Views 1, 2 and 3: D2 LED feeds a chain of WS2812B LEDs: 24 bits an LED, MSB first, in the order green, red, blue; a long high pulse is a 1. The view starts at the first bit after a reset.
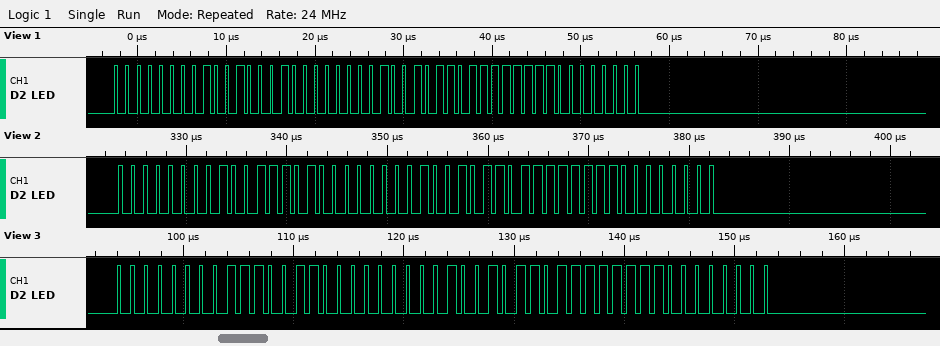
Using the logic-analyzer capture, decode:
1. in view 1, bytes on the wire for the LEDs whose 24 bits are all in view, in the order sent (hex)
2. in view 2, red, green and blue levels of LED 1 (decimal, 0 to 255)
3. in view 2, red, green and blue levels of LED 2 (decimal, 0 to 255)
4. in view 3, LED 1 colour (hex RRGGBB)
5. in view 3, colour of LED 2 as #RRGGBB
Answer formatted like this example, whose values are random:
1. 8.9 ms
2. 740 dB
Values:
1. 00 91 00 96 FF 00
2. 157, 0, 0
3. 255, 150, 0
4. #E60000
5. #FF9600
